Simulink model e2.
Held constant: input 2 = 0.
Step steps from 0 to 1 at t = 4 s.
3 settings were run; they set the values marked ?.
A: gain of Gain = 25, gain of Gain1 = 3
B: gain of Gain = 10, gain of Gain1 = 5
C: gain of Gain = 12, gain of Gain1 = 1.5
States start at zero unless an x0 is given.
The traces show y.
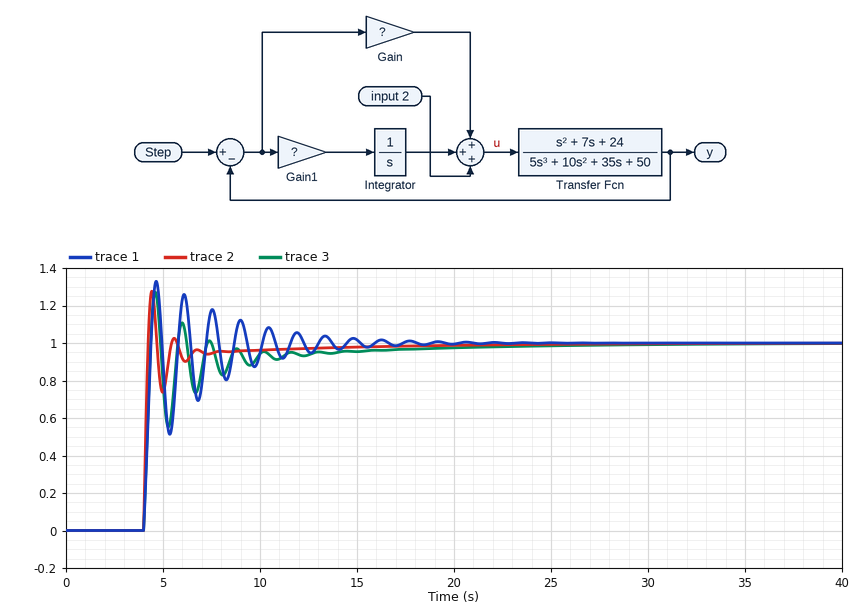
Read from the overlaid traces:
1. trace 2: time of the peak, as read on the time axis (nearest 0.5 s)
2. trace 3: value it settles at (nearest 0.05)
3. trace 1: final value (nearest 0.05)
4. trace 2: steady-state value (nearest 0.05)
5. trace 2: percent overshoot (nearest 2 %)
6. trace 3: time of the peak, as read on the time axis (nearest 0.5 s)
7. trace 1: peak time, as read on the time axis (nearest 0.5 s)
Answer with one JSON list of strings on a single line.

["4.5 s", "1.00", "1.00", "1.00", "28 %", "4.5 s", "4.5 s"]
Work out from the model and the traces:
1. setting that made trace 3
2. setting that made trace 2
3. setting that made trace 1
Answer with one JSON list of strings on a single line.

["C", "A", "B"]
